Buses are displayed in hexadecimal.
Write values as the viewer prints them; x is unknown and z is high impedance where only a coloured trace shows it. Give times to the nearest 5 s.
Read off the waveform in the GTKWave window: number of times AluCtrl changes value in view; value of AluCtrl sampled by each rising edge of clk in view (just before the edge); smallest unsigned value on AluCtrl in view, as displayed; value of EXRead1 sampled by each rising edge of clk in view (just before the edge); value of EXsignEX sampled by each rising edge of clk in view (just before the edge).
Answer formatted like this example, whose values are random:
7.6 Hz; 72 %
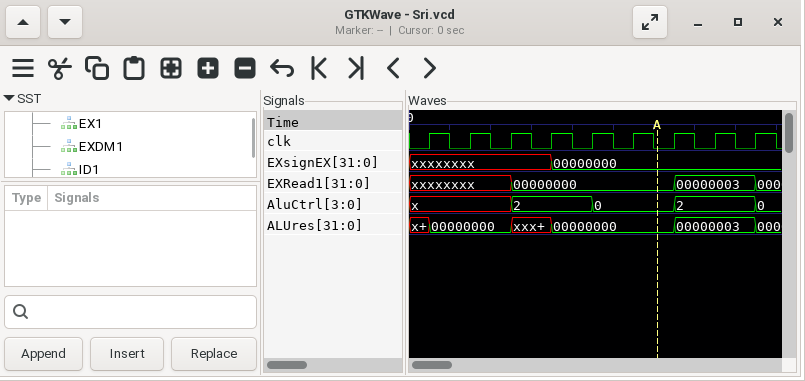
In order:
4; x, x, x, 2, 2, 0, 0, 2, 2; 0; xxxxxxxx, xxxxxxxx, xxxxxxxx, 00000000, 00000000, 00000000, 00000000, 00000003, 00000003; xxxxxxxx, xxxxxxxx, xxxxxxxx, xxxxxxxx, 00000000, 00000000, 00000000, 00000000, 00000000
